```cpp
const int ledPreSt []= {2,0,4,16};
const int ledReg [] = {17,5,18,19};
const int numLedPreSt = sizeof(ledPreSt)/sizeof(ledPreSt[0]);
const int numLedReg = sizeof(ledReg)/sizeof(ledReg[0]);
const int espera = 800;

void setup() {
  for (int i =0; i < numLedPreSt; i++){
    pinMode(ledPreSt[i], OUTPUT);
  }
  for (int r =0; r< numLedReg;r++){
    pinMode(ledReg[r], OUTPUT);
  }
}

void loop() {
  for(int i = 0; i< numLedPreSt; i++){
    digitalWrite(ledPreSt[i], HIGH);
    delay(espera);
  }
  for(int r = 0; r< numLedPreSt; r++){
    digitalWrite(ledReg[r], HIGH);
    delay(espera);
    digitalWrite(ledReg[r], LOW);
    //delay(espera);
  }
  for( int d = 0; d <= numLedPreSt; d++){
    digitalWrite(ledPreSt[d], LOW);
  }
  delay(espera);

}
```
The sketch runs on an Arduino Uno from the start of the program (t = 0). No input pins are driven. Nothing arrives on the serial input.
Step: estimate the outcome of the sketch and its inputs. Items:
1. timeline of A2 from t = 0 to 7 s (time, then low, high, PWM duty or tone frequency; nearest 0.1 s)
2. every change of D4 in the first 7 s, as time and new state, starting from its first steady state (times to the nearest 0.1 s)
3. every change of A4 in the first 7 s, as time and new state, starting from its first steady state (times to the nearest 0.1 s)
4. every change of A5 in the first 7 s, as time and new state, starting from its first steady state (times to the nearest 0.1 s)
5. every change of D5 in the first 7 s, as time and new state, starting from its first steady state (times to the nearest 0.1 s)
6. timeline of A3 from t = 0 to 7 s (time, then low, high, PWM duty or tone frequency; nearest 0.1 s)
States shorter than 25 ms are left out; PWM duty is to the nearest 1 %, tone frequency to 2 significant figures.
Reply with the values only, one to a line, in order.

0 s low; 2.4 s high; 6.4 s low
0 s low; 1.6 s high; 6.4 s low
0 s low; 4.8 s high; 5.6 s low
0 s low; 5.6 s high; 6.4 s low
0 s low; 4 s high; 4.8 s low
0 s low; 3.2 s high; 4 s low
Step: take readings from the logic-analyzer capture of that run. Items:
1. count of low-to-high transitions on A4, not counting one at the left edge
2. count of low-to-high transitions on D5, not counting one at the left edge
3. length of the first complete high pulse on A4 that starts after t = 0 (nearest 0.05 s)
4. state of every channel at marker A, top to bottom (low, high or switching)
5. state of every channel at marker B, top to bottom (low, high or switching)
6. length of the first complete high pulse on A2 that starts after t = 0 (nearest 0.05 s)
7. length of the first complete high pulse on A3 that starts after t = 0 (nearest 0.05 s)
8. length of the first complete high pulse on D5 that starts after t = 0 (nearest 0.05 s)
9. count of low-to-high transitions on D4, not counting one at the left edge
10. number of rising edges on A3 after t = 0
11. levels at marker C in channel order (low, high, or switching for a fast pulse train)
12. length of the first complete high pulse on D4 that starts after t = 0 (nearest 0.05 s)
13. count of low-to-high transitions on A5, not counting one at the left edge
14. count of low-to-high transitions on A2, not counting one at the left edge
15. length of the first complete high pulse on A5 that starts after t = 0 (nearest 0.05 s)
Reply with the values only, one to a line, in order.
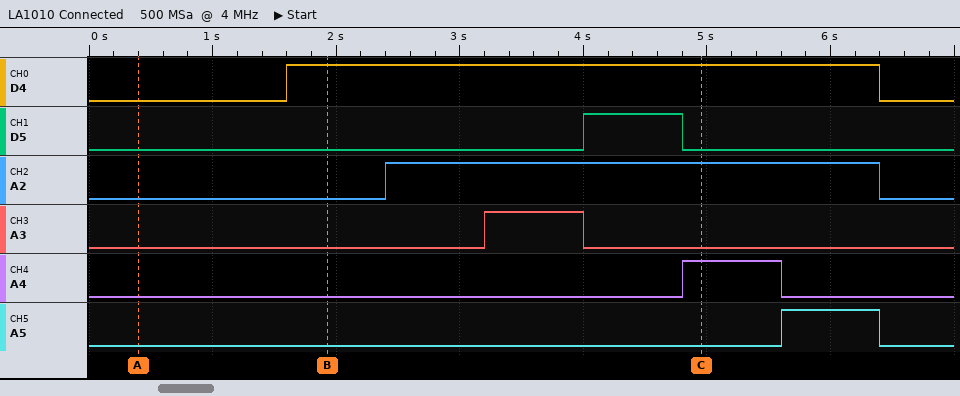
1
1
0.80 s
D4 low, D5 low, A2 low, A3 low, A4 low, A5 low
D4 high, D5 low, A2 low, A3 low, A4 low, A5 low
4.00 s
0.80 s
0.80 s
1
1
D4 high, D5 low, A2 high, A3 low, A4 high, A5 low
4.80 s
1
1
0.80 s
